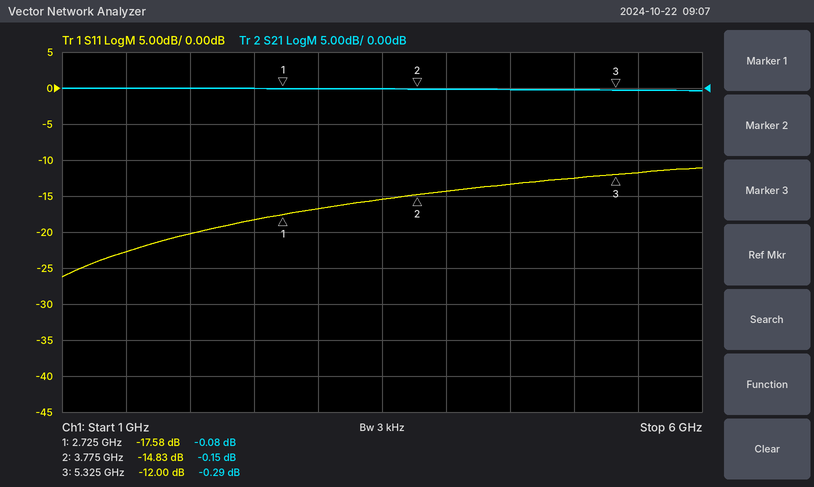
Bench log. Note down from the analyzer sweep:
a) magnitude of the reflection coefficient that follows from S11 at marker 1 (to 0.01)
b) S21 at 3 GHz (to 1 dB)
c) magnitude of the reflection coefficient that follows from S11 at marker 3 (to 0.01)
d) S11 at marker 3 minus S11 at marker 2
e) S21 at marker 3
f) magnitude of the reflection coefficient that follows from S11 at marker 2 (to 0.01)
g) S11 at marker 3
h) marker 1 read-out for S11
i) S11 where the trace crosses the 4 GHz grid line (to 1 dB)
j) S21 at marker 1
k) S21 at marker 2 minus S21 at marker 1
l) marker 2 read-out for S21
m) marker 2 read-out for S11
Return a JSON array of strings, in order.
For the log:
["0.13", "0 dB", "0.25", "2.83 dB", "-0.29 dB", "0.18", "-12.00 dB", "-17.58 dB", "-14 dB", "-0.08 dB", "-0.07 dB", "-0.15 dB", "-14.83 dB"]
